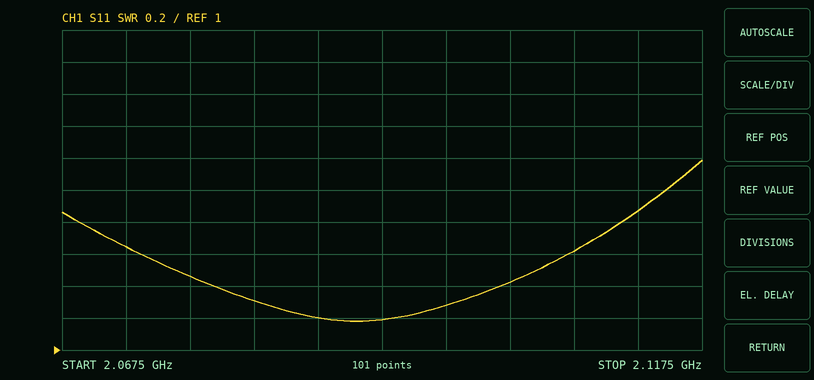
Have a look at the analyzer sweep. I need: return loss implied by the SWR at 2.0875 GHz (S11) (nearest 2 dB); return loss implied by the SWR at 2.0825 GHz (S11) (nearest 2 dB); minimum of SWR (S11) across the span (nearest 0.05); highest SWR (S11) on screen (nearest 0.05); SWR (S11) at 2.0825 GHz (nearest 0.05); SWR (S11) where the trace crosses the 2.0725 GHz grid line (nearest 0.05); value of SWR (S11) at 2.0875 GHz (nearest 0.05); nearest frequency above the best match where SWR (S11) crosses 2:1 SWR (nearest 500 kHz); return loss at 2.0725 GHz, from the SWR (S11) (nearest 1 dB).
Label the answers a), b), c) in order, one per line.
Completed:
a) 20 dB
b) 18 dB
c) 1.20
d) 2.20
e) 1.30
f) 1.65
g) 1.20
h) 2.1145 GHz
i) 12 dB
